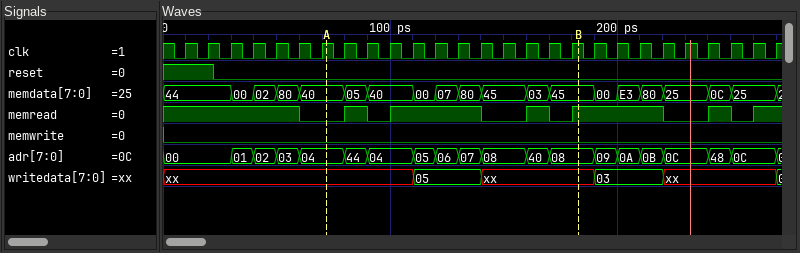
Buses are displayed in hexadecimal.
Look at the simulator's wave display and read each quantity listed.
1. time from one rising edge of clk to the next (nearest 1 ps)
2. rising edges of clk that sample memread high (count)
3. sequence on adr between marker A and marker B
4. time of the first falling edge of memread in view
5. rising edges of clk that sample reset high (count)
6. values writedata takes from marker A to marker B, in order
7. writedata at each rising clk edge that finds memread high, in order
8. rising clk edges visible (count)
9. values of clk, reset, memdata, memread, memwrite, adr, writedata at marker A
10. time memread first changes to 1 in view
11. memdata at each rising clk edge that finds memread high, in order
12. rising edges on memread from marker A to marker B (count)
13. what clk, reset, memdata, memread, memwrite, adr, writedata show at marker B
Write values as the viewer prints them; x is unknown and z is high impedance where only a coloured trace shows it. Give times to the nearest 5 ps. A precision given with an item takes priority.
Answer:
10 ps
18
04, 44, 04, 05, 06, 07, 08, 40, 08
60 ps
2
xx, 05, xx
xx, xx, xx, xx, xx, xx, xx, xx, 05, 05, 05, xx, xx, 03, 03, 03, xx, xx
27
clk=1, reset=0, memdata=40, memread=0, memwrite=0, adr=04, writedata=xx
80 ps
44, 44, 44, 00, 02, 80, 05, 40, 00, 07, 80, 03, 45, 00, E3, 80, 0C, 25
4
clk=1, reset=0, memdata=45, memread=1, memwrite=0, adr=08, writedata=xx
